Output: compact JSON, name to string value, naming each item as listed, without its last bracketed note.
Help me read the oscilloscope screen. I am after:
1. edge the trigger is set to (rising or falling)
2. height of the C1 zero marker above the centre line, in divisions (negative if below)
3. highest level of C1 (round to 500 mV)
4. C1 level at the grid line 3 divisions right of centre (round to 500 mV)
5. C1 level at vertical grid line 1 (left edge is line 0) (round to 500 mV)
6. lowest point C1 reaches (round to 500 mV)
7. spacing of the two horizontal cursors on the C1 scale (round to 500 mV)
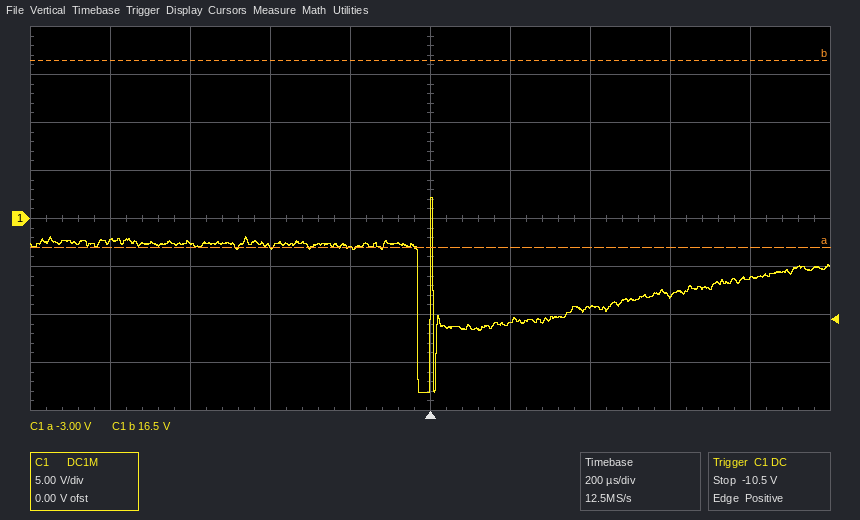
{"edge the trigger is set to": "rising", "height of the C1 zero marker above the centre line, in divisions": "0.0 div", "highest level of C1": "2.0 V", "C1 level at the grid line 3 divisions right of centre": "-8.0 V", "C1 level at vertical grid line 1 (left edge is line 0)": "-2.5 V", "lowest point C1 reaches": "-18.0 V", "spacing of the two horizontal cursors on the C1 scale": "19.5 V"}
